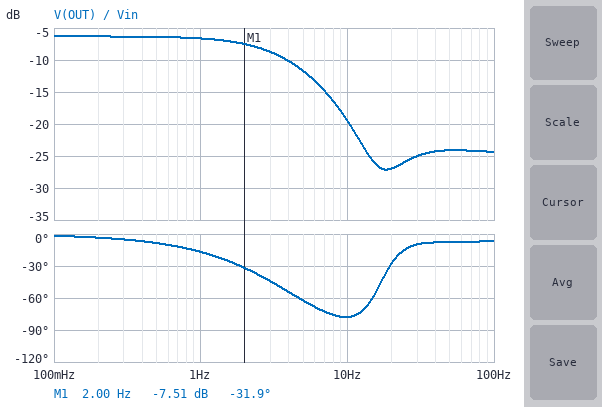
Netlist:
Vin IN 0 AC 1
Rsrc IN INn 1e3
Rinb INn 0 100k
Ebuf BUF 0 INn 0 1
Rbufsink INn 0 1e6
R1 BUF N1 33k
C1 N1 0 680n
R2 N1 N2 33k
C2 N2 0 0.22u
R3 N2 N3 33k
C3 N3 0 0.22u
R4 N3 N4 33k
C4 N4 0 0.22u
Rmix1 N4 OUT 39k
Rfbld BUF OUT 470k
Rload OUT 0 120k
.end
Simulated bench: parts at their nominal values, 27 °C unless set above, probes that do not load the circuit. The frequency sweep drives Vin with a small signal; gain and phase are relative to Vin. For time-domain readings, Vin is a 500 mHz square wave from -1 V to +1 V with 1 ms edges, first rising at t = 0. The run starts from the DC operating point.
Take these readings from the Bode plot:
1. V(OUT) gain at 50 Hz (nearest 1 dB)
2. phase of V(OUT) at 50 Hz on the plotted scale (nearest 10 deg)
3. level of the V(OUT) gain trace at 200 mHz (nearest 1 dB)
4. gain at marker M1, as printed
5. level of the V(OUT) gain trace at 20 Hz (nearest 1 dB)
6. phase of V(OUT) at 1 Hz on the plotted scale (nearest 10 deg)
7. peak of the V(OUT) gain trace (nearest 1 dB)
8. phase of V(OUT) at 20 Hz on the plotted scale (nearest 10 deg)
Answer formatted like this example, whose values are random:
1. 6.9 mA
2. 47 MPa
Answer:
1. -24 dB
2. -10 deg
3. -6 dB
4. -7.51 dB
5. -27 dB
6. -20 deg
7. -6 dB
8. -30 deg
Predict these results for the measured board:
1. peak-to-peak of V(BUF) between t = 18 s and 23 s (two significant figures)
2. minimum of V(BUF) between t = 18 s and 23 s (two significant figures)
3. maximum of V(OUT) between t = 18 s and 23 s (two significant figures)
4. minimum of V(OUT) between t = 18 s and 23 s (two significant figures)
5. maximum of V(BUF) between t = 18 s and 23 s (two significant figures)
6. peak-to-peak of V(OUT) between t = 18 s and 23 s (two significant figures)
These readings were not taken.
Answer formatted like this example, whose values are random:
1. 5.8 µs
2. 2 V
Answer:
1. 2.0 V
2. -990 mV
3. 480 mV
4. -480 mV
5. 990 mV
6. 970 mV
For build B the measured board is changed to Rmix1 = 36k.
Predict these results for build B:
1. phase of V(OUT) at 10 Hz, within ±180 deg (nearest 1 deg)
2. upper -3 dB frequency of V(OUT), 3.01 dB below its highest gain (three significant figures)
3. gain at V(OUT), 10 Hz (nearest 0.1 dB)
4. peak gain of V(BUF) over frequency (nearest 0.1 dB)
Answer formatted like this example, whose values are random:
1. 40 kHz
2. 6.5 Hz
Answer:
1. -80 deg
2. 3.43 Hz
3. -19.3 dB
4. -0.1 dB
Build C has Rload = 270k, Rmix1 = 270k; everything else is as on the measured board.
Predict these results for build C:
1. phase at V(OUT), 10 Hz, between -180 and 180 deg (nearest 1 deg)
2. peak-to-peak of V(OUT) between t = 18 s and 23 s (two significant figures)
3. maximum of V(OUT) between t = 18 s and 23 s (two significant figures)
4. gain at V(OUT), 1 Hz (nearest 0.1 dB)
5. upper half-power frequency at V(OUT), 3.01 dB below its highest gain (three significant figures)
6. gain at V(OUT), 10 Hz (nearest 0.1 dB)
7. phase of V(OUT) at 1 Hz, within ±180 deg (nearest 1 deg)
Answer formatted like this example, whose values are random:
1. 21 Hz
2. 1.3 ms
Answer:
1. -16 deg
2. 1.1 V
3. 550 mV
4. -5.7 dB
5. 2.80 Hz
6. -14.4 dB
7. -15 deg
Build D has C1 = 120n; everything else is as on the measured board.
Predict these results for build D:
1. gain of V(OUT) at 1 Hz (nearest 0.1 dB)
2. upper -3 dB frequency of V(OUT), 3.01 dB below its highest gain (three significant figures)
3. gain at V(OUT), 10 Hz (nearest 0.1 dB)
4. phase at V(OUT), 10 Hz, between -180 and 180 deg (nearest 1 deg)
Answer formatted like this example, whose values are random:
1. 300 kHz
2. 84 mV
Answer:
1. -6.5 dB
2. 4.51 Hz
3. -15.0 dB
4. -70 deg
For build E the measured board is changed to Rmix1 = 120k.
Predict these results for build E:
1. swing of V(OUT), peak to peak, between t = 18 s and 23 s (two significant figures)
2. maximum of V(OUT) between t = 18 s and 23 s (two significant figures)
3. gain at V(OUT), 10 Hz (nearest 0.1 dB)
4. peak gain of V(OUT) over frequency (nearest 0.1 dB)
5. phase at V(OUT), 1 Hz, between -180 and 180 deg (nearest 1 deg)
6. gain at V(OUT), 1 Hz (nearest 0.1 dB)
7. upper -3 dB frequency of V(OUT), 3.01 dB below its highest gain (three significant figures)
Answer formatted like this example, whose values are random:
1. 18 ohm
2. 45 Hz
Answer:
1. 840 mV
2. 420 mV
3. -20.2 dB
4. -7.6 dB
5. -16 deg
6. -8.0 dB
7. 3.01 Hz
